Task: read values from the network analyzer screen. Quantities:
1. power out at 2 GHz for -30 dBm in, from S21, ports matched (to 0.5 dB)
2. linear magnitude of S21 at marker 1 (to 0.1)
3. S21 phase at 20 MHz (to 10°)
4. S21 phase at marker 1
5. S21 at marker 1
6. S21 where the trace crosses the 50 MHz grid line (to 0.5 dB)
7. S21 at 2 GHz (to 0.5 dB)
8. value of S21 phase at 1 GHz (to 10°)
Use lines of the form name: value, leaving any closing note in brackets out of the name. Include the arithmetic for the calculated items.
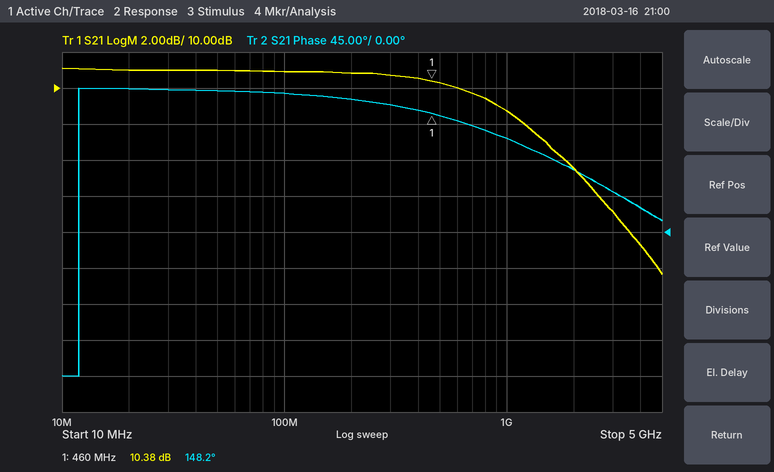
power out at 2 GHz for -30 dBm in, from S21, ports matched: -30 dBm + (5.5 dB) = -24.5 dBm
linear magnitude of S21 at marker 1: 10^(10.38/20) ≈ 3.3
S21 phase at 20 MHz: 180°
S21 phase at marker 1: 148.2°
S21 at marker 1: 10.38 dB
S21 where the trace crosses the 50 MHz grid line: 11.0 dB
S21 at 2 GHz: 5.5 dB
value of S21 phase at 1 GHz: 120°
